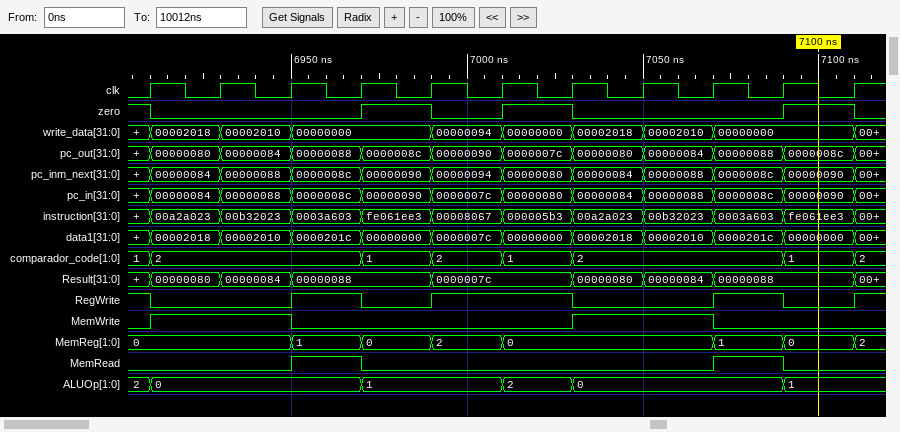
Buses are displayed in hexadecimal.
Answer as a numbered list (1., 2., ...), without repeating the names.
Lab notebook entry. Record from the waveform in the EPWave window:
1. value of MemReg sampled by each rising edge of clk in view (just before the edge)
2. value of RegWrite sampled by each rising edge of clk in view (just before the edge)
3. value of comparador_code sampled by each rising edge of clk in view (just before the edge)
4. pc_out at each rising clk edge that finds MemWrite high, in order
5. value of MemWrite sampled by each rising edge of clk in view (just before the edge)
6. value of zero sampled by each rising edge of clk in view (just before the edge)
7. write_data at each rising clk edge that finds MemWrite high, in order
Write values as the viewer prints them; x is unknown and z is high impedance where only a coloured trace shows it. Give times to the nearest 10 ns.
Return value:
1. 0, 0, 0, 1, 0, 2, 0, 0, 0, 1, 0
2. 1 0 0 1 0 1 1 0 0 1 0
3. 1, 2, 2, 2, 1, 2, 1, 2, 2, 2, 1
4. 00000080, 00000084, 00000080, 00000084
5. 0 1 1 0 0 0 0 1 1 0 0
6. 1 0 0 0 1 0 1 0 0 0 1
7. 00002018, 00002010, 00002018, 00002010
